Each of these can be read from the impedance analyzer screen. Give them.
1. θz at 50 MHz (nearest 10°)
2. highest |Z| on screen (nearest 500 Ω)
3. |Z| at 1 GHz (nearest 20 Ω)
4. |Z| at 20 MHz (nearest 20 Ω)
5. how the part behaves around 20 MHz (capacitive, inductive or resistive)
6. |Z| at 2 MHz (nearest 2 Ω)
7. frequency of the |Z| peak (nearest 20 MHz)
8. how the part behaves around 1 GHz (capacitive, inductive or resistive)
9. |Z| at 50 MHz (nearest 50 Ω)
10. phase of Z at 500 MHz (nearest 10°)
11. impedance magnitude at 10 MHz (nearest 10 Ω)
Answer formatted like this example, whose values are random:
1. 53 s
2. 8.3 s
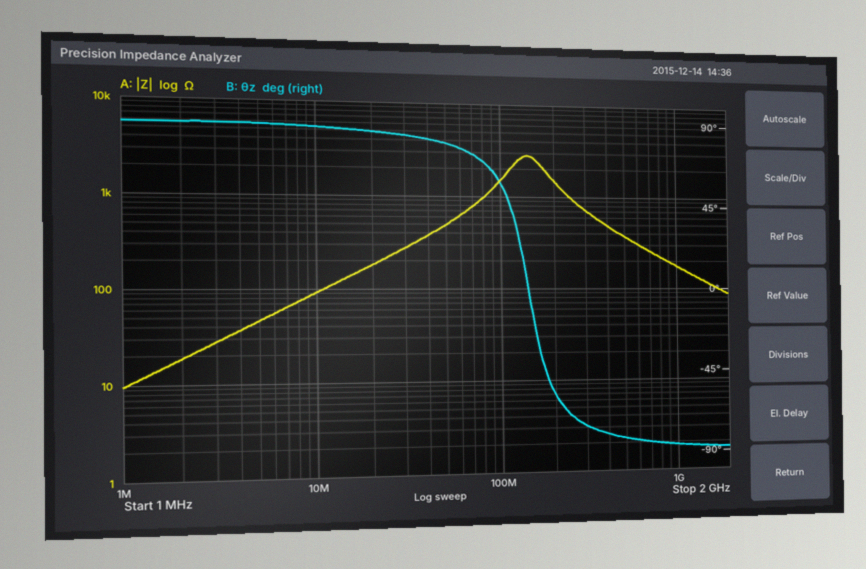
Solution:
1. 80°
2. 3.0 kΩ
3. 180 Ω
4. 180 Ω
5. inductive
6. 18 Ω
7. 140 MHz
8. capacitive
9. 500 Ω
10. -80°
11. 90 Ω
